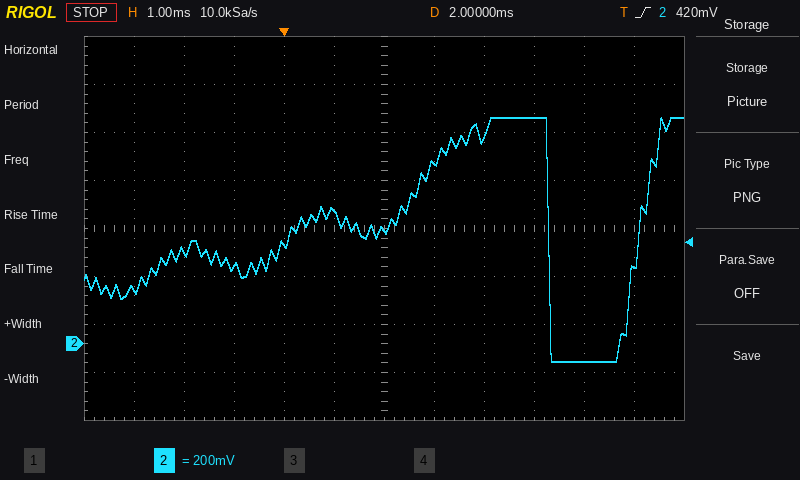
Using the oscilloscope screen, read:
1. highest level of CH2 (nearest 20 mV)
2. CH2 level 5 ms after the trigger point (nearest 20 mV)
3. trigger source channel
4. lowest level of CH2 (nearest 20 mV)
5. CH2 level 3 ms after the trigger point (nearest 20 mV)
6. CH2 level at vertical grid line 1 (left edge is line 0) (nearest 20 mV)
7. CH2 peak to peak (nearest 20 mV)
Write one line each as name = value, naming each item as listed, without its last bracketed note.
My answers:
highest level of CH2 = 940 mV
CH2 level 5 ms after the trigger point = 940 mV
trigger source channel = CH2
lowest level of CH2 = -80 mV
CH2 level 3 ms after the trigger point = 760 mV
CH2 level at vertical grid line 1 (left edge is line 0) = 220 mV
CH2 peak to peak = 1.02 V
